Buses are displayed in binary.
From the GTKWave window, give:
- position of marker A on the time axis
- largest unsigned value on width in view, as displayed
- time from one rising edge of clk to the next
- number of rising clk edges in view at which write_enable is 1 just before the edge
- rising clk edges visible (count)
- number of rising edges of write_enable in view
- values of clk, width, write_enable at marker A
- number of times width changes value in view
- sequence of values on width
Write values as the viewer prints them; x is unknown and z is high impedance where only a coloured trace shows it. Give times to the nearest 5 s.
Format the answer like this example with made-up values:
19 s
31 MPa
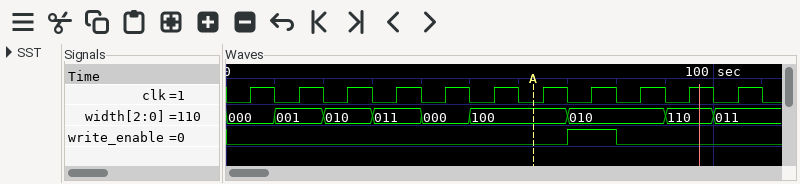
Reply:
65 s
110
10 s
1
11
1
clk=0, width=100, write_enable=0
8
000, 001, 010, 011, 000, 100, 010, 110, 011
